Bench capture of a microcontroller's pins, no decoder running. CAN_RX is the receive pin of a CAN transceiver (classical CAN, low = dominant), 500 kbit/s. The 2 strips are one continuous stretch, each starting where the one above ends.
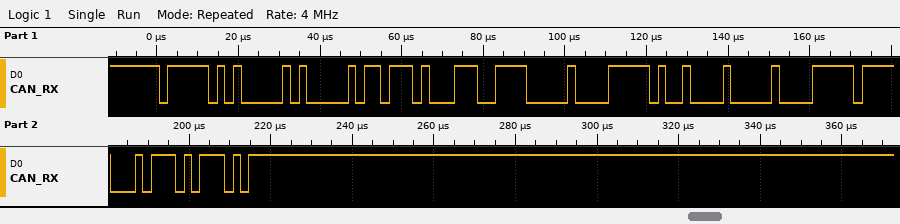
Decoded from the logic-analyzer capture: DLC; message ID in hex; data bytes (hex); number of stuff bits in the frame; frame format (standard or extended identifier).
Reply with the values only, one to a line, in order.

8
0x7E8
1B A3 9E 00 FC 84 01 FF
7
standard
